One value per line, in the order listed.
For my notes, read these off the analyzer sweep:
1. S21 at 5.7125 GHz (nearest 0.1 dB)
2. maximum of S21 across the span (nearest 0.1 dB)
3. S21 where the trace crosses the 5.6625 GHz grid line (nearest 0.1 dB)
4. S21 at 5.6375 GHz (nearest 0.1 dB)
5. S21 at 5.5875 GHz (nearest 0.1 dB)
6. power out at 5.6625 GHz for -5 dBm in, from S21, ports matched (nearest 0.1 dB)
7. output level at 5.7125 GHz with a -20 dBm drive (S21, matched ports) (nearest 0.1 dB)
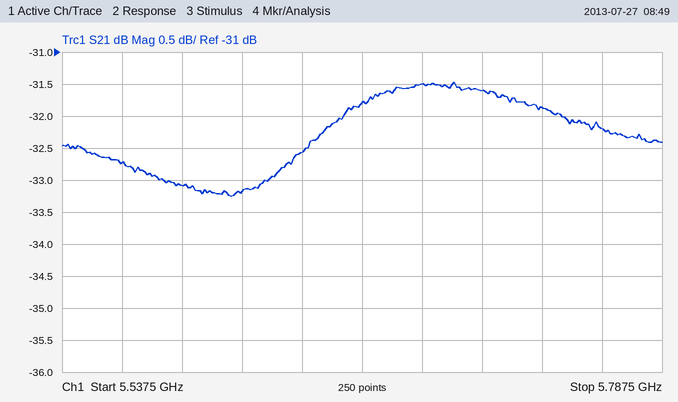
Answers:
-31.6 dB
-31.5 dB
-31.8 dB
-32.6 dB
-33.1 dB
-36.8 dBm
-51.6 dBm
